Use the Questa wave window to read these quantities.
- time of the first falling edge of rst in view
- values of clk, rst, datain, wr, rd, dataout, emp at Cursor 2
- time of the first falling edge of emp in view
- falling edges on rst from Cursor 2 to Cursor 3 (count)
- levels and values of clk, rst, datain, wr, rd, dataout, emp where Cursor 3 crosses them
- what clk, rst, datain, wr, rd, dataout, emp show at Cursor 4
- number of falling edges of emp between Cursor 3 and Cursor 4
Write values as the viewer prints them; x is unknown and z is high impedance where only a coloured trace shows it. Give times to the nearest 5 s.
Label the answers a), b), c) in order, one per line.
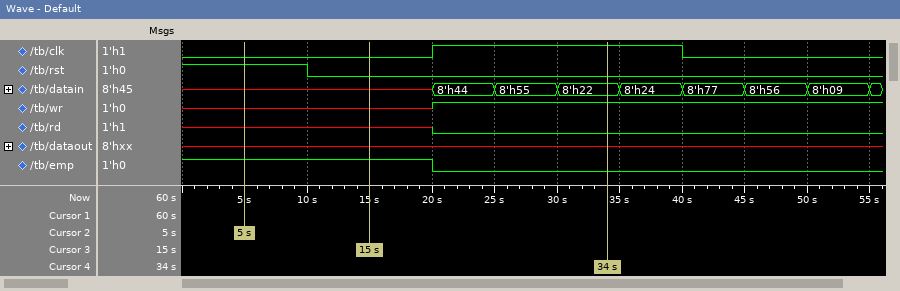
a) 10 s
b) clk=0, rst=1, datain=x, wr=x, rd=x, dataout=x, emp=1
c) 20 s
d) 1
e) clk=0, rst=0, datain=x, wr=x, rd=x, dataout=x, emp=1
f) clk=1, rst=0, datain=8'h22, wr=1, rd=0, dataout=x, emp=0
g) 1
